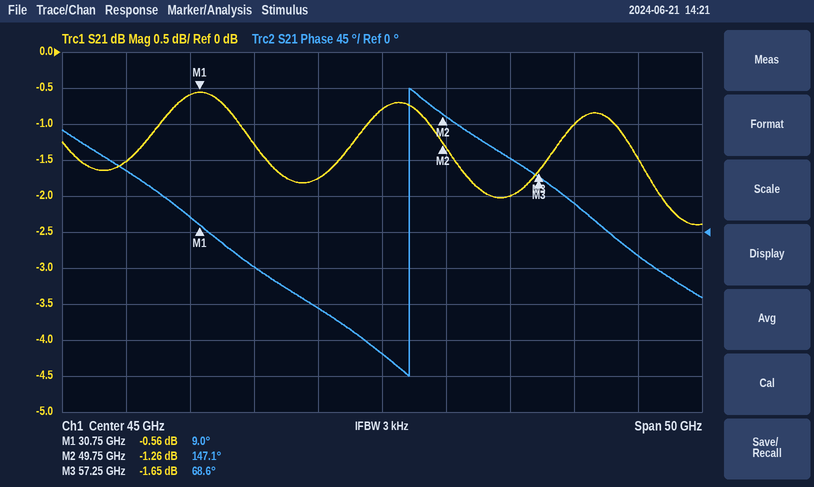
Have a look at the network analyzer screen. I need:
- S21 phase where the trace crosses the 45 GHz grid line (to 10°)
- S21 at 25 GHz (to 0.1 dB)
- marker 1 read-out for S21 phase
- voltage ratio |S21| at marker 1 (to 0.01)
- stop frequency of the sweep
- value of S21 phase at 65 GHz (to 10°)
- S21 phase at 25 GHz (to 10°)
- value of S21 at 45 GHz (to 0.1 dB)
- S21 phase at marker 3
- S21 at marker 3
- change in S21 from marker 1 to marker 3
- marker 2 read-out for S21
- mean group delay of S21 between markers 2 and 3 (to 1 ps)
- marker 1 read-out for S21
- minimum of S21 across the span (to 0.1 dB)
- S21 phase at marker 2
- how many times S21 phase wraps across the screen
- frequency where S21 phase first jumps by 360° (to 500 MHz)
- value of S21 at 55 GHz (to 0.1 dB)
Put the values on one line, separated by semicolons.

-150°; -1.5 dB; 9.0°; 0.94; 70 GHz; -30°; 80°; -0.8 dB; 68.6°; -1.65 dB; -1.09 dB; -1.26 dB; 29 ps; -0.56 dB; -2.4 dB; 147.1°; 1; 47.0 GHz; -2.0 dB
